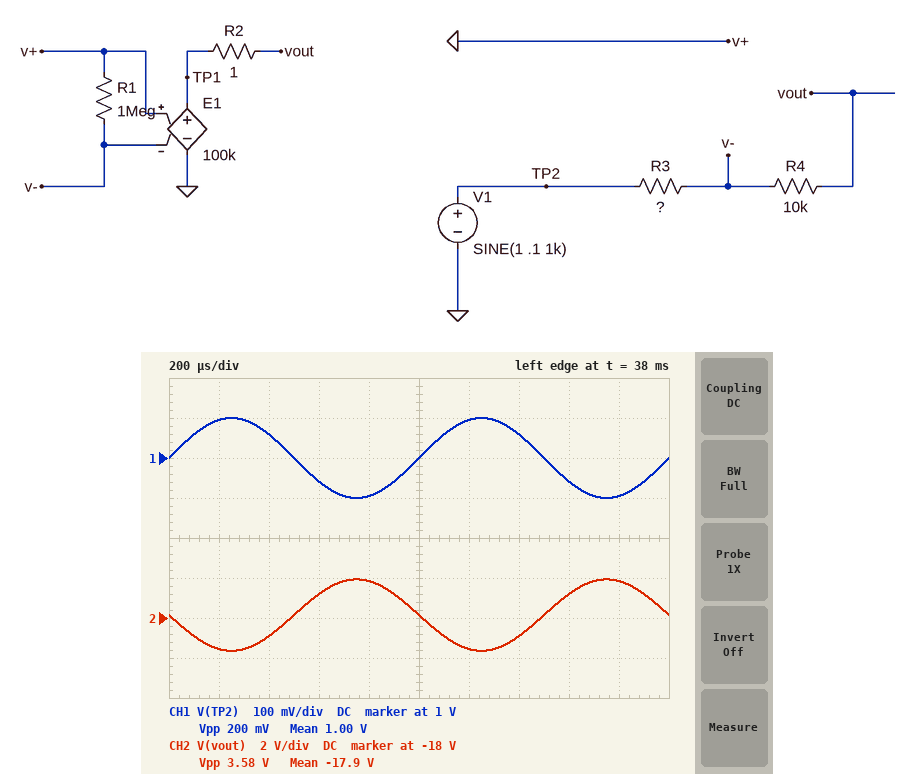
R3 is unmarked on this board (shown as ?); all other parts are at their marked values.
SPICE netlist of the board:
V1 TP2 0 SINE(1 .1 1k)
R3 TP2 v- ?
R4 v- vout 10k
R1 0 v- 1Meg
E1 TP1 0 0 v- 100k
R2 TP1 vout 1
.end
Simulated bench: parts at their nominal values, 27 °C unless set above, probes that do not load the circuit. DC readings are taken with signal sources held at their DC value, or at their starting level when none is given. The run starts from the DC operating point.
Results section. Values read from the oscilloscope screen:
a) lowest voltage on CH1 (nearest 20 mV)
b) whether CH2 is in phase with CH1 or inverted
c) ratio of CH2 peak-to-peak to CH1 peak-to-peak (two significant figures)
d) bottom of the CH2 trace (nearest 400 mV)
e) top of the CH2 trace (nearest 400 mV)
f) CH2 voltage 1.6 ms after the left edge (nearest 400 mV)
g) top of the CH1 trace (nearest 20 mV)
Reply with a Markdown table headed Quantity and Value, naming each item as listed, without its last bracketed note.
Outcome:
| Quantity | Value |
|---|---|
| lowest voltage on CH1 | 900 mV |
| whether CH2 is in phase with CH1 or inverted | inverted |
| ratio of CH2 peak-to-peak to CH1 peak-to-peak | 18 |
| bottom of the CH2 trace | -19.6 V |
| top of the CH2 trace | -16.0 V |
| CH2 voltage 1.6 ms after the left edge | -16.8 V |
| top of the CH1 trace | 1.10 V |
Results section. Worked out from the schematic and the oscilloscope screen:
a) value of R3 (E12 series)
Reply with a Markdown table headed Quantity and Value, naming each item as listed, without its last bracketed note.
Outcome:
| Quantity | Value |
|---|---|
| value of R3 | 560 Ω |
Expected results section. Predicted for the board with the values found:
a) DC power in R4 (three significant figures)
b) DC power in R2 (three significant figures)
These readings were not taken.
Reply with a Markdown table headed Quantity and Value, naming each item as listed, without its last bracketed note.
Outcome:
| Quantity | Value |
|---|---|
| DC power in R4 | 31.9 mW |
| DC power in R2 | 3.19 µW |
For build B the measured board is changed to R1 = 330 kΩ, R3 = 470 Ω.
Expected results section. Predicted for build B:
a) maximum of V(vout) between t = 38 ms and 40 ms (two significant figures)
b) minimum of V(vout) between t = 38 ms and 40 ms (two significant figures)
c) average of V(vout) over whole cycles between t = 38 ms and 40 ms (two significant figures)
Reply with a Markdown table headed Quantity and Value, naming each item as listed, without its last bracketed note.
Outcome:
| Quantity | Value |
|---|---|
| maximum of V(vout) between t = 38 ms and 40 ms | -19 V |
| minimum of V(vout) between t = 38 ms and 40 ms | -23 V |
| average of V(vout) over whole cycles between t = 38 ms and 40 ms | -21 V |
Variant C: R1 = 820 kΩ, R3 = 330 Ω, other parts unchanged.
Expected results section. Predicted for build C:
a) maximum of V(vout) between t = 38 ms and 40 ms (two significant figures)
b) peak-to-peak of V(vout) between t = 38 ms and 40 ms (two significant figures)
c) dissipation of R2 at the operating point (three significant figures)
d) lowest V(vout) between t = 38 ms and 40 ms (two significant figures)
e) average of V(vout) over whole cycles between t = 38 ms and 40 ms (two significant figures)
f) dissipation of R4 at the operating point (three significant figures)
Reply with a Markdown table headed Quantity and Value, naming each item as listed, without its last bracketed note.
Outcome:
| Quantity | Value |
|---|---|
| maximum of V(vout) between t = 38 ms and 40 ms | -27 V |
| peak-to-peak of V(vout) between t = 38 ms and 40 ms | 6.1 V |
| dissipation of R2 at the operating point | 9.18 µW |
| lowest V(vout) between t = 38 ms and 40 ms | -33 V |
| average of V(vout) over whole cycles between t = 38 ms and 40 ms | -30 V |
| dissipation of R4 at the operating point | 91.8 mW |
